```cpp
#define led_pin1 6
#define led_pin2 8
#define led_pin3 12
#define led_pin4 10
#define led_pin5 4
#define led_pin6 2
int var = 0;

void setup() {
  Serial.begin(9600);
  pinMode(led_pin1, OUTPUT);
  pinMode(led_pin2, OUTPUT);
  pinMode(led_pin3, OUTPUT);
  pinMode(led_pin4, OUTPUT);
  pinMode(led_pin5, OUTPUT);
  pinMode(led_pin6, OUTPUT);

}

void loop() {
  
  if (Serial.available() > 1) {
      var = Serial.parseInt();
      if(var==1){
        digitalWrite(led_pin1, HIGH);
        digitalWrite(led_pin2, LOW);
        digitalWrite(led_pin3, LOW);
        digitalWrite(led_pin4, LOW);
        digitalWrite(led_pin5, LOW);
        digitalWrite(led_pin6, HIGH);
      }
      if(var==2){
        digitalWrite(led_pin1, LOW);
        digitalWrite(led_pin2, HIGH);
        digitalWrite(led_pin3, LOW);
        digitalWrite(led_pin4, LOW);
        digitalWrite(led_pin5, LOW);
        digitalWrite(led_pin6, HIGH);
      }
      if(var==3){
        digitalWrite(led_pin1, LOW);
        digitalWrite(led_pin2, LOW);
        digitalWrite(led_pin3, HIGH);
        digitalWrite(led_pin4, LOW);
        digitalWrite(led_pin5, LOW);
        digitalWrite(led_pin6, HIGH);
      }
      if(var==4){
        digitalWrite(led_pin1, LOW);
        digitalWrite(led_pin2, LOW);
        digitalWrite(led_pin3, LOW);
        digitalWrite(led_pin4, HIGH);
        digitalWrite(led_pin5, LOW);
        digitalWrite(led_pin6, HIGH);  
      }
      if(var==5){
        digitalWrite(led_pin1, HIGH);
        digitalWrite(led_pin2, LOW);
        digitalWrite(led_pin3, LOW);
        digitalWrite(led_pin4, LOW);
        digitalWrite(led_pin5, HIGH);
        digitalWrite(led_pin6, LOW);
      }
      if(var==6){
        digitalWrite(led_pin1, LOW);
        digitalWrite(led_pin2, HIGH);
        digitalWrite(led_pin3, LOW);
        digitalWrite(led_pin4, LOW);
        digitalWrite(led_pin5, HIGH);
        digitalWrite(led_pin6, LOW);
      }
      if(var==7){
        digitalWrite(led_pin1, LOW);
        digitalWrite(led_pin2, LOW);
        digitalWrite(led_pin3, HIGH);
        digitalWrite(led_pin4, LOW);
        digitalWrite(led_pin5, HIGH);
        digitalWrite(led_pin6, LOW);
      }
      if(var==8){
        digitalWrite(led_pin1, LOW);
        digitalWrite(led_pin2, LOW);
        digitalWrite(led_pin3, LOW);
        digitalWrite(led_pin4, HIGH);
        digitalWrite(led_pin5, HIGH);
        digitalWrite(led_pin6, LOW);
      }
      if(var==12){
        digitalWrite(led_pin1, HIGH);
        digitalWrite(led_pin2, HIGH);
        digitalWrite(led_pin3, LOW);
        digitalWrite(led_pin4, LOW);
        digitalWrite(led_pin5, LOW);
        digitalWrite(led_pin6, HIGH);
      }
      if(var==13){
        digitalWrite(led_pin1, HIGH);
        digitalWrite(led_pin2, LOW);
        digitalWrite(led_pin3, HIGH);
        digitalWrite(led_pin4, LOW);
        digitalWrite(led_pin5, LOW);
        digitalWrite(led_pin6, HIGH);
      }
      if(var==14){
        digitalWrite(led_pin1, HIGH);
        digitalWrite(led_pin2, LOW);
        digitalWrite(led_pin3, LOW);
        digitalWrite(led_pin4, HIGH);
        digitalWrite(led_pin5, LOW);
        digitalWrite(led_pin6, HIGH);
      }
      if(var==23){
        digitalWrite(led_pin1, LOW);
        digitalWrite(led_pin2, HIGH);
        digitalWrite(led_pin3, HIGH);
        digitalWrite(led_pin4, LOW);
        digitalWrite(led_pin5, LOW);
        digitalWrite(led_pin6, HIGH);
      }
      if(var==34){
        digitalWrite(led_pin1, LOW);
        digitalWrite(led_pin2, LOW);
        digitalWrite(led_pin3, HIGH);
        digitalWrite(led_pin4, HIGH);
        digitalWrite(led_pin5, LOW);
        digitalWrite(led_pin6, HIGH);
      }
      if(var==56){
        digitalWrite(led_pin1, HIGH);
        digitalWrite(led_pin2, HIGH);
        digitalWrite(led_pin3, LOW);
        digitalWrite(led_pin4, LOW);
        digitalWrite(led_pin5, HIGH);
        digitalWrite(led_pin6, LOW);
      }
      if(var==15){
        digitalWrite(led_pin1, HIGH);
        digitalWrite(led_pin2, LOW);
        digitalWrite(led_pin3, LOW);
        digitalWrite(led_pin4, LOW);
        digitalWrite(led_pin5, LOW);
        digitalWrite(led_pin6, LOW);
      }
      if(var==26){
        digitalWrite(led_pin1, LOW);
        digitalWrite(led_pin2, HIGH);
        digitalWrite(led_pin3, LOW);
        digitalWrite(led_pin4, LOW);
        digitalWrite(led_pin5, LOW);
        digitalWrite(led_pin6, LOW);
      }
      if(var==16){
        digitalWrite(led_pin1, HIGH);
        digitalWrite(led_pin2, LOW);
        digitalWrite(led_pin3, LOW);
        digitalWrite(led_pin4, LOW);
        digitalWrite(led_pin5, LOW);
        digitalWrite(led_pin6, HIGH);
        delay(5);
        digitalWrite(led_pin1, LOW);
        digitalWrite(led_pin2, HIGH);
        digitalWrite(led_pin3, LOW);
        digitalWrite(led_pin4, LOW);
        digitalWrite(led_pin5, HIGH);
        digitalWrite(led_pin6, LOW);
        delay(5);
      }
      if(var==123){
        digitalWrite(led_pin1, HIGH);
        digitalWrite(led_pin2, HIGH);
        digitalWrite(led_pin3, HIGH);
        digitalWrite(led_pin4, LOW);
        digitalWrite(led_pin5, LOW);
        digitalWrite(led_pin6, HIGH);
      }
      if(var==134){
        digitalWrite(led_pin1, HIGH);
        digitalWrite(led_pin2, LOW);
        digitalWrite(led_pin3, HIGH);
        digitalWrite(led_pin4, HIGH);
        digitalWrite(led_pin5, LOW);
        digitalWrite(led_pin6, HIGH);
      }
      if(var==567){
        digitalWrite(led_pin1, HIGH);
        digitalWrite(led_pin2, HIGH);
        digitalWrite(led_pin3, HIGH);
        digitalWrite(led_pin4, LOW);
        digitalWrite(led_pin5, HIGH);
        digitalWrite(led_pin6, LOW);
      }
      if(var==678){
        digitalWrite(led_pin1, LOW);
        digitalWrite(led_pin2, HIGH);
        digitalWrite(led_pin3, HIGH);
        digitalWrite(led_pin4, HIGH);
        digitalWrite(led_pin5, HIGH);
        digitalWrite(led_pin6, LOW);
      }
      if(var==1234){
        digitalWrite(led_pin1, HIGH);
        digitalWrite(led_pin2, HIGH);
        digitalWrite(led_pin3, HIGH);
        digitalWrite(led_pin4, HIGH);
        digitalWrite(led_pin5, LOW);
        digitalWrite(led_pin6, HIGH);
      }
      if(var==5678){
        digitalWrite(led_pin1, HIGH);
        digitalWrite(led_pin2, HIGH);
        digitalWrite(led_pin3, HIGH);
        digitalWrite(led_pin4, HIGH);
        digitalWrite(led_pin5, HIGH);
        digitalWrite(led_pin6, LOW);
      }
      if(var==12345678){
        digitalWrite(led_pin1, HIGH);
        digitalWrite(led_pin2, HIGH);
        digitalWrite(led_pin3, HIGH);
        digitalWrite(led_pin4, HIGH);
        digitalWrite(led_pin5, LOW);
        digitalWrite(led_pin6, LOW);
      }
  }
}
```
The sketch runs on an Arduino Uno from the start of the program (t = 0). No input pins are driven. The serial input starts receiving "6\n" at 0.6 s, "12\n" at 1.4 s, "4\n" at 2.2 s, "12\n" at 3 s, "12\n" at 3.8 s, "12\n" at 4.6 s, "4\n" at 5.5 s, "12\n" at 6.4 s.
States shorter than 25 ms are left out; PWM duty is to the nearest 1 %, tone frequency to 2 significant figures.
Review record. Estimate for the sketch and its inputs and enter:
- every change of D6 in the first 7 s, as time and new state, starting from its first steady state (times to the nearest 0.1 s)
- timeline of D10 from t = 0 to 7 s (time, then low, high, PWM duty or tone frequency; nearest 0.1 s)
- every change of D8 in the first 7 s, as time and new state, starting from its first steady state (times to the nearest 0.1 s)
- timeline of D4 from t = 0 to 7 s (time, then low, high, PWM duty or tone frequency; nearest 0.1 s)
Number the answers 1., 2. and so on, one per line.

1. 0 s low; 1.4 s high; 2.2 s low; 3 s high; 5.5 s low; 6.4 s high
2. 0 s low; 2.2 s high; 3 s low; 5.5 s high; 6.4 s low
3. 0 s low; 0.6 s high; 2.2 s low; 3 s high; 5.5 s low; 6.4 s high
4. 0 s low; 0.6 s high; 1.4 s low
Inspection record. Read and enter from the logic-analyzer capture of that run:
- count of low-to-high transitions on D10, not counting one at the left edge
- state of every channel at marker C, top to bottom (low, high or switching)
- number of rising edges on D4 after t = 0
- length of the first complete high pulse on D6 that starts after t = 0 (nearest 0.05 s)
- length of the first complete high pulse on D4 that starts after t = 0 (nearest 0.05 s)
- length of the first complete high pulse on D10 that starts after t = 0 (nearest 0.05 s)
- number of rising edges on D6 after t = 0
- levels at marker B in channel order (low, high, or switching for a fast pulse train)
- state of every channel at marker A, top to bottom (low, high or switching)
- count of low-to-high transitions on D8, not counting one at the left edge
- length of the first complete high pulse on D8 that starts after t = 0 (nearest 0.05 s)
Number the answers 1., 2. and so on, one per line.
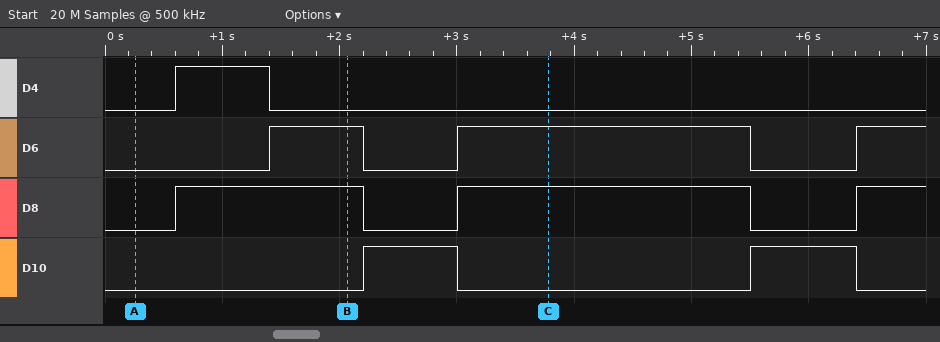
1. 2
2. D4 low, D6 high, D8 high, D10 low
3. 1
4. 0.80 s
5. 0.80 s
6. 0.80 s
7. 3
8. D4 low, D6 high, D8 high, D10 low
9. D4 low, D6 low, D8 low, D10 low
10. 3
11. 1.60 s
